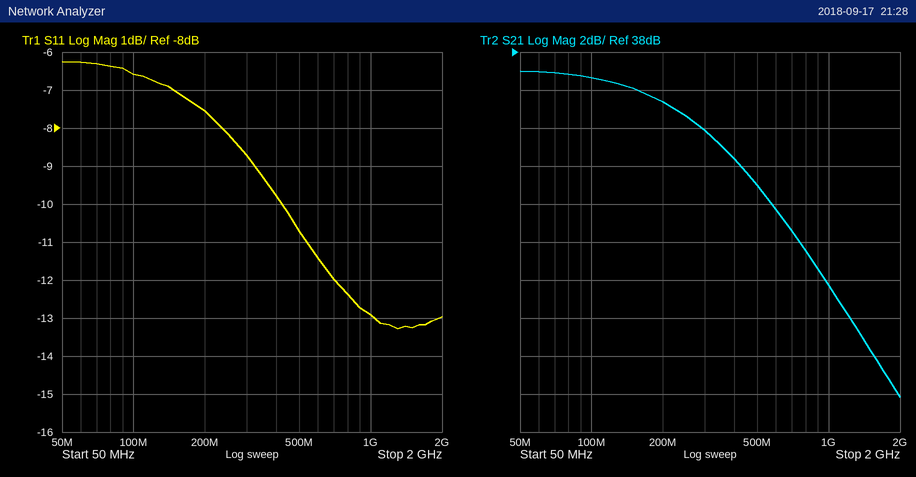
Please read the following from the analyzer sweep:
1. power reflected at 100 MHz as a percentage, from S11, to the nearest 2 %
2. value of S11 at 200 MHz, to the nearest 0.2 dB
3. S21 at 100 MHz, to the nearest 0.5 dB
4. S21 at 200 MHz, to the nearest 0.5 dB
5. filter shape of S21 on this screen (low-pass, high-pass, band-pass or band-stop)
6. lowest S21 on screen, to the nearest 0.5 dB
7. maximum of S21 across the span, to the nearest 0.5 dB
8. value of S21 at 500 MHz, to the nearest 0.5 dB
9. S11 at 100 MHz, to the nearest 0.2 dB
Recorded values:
22 %
-7.6 dB
36.5 dB
35.5 dB
low-pass
20.0 dB
37.0 dB
31.0 dB
-6.6 dB
